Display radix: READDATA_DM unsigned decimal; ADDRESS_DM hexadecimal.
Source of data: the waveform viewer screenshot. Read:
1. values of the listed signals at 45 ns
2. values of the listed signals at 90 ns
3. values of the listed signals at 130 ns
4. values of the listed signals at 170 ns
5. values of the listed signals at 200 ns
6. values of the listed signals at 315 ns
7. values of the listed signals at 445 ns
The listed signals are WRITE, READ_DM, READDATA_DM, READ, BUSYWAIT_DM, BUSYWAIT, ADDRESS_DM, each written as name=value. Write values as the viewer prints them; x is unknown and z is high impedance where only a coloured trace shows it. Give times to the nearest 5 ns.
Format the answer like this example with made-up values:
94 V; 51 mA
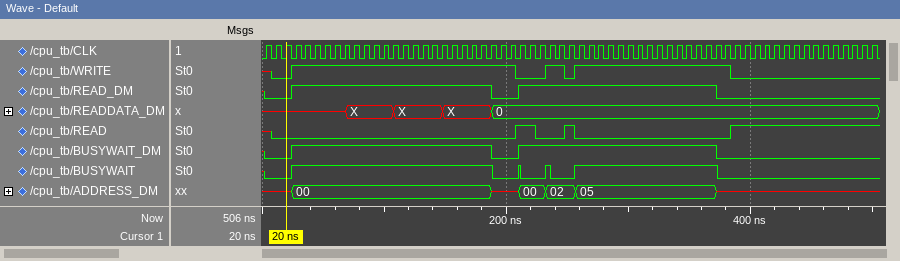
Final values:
WRITE=1, READ_DM=1, READDATA_DM=x, READ=0, BUSYWAIT_DM=1, BUSYWAIT=1, ADDRESS_DM=00; WRITE=1, READ_DM=1, READDATA_DM=X, READ=0, BUSYWAIT_DM=1, BUSYWAIT=1, ADDRESS_DM=00; WRITE=1, READ_DM=1, READDATA_DM=X, READ=0, BUSYWAIT_DM=1, BUSYWAIT=1, ADDRESS_DM=00; WRITE=1, READ_DM=1, READDATA_DM=X, READ=0, BUSYWAIT_DM=1, BUSYWAIT=1, ADDRESS_DM=00; WRITE=1, READ_DM=0, READDATA_DM=0, READ=0, BUSYWAIT_DM=0, BUSYWAIT=0, ADDRESS_DM=x; WRITE=1, READ_DM=1, READDATA_DM=0, READ=0, BUSYWAIT_DM=1, BUSYWAIT=1, ADDRESS_DM=05; WRITE=0, READ_DM=0, READDATA_DM=0, READ=1, BUSYWAIT_DM=0, BUSYWAIT=0, ADDRESS_DM=x
